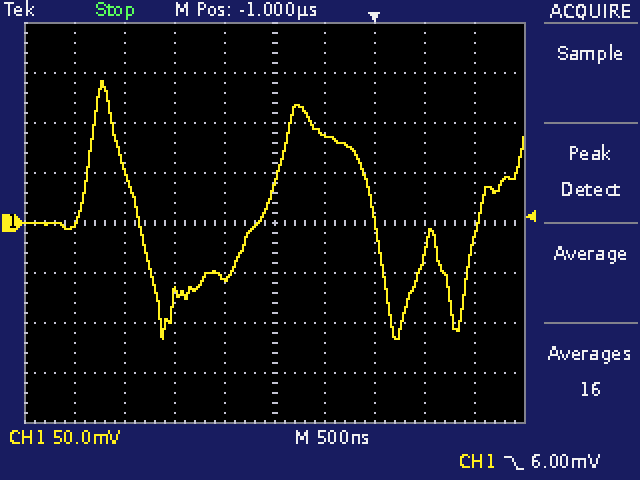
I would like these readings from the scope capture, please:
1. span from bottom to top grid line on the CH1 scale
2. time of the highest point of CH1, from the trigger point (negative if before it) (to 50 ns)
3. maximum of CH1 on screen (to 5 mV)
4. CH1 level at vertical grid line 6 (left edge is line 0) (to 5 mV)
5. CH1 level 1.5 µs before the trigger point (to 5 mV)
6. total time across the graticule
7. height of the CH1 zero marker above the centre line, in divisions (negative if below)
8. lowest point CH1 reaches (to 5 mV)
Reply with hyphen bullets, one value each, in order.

- 400 mV
- -2.70 µs
- 140 mV
- 90 mV
- -55 mV
- 5 µs
- 0.0 div
- -115 mV
